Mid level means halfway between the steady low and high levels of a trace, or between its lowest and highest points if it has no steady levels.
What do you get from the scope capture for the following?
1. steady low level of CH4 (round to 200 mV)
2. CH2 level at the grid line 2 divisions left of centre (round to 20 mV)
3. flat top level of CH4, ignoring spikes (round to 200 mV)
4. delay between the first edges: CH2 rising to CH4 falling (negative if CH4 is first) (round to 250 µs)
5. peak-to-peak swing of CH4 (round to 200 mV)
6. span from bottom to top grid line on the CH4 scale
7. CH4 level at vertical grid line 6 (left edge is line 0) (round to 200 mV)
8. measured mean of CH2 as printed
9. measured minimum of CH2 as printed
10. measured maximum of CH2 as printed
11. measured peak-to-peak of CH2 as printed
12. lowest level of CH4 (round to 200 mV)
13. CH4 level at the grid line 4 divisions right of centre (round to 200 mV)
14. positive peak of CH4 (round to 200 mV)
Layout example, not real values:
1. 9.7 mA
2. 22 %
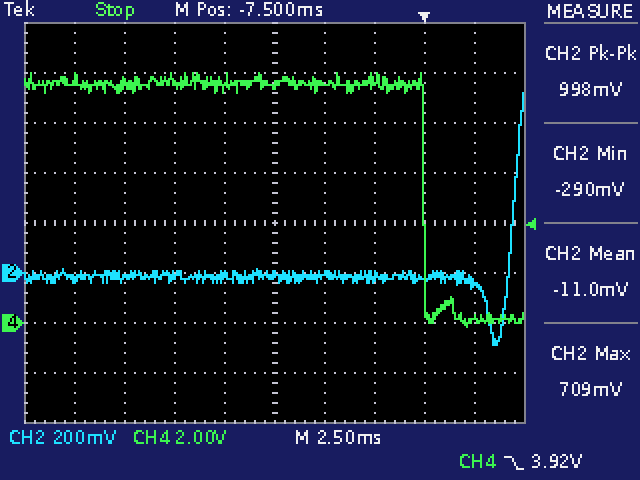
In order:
1. 200 mV
2. -20 mV
3. 9.6 V
4. -4.50 ms
5. 10.2 V
6. 16 V
7. 9.6 V
8. -11.0 mV
9. -290 mV
10. 709 mV
11. 998 mV
12. -200 mV
13. 200 mV
14. 10.0 V
